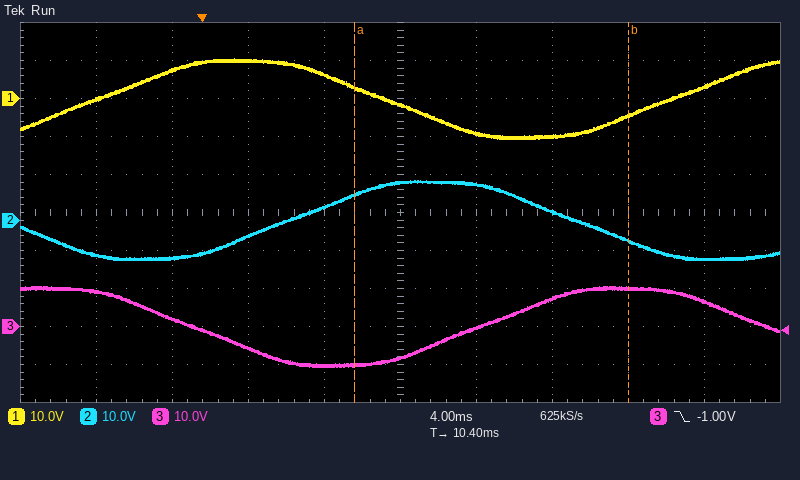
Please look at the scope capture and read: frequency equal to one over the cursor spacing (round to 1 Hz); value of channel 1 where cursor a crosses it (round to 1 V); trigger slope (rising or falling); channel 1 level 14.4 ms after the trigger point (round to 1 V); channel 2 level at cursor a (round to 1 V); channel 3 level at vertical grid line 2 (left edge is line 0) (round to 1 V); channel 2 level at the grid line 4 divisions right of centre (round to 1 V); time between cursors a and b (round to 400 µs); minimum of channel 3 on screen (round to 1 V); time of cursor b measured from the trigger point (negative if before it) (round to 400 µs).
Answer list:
69 Hz
3 V
falling
-9 V
7 V
2 V
-10 V
14.4 ms
-11 V
+22.4 ms
